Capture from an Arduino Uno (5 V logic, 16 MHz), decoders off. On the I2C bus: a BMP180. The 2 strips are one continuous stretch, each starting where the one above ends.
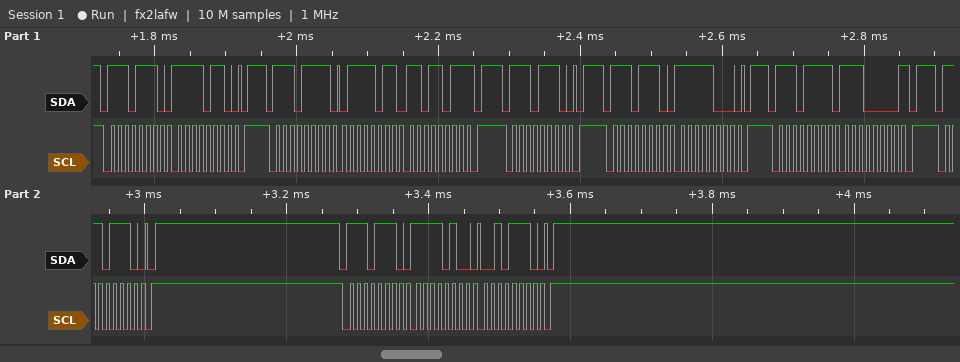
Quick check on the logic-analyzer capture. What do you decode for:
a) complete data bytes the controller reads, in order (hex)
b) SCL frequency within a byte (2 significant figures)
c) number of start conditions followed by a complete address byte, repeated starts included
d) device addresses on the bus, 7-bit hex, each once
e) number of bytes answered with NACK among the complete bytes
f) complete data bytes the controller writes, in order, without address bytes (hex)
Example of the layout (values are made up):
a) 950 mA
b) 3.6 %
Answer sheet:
a) 7B DB E0
b) 100 kHz
c) 7
d) 0x77
e) 2
f) F6 F8 F4 2E
